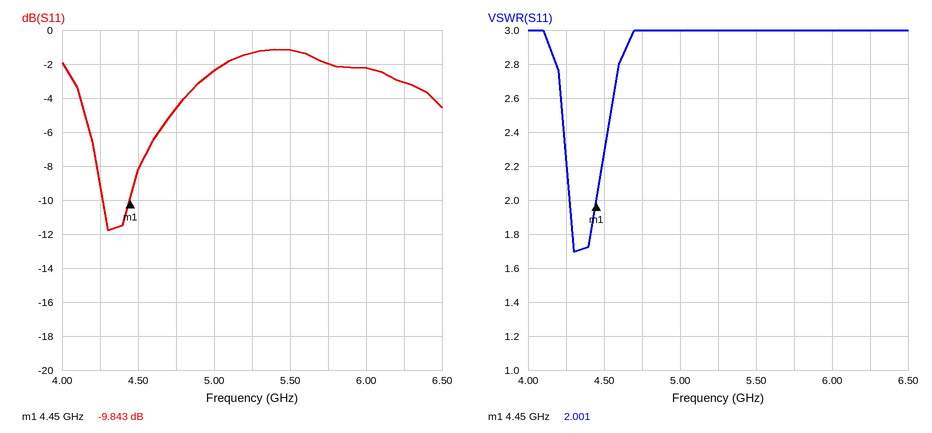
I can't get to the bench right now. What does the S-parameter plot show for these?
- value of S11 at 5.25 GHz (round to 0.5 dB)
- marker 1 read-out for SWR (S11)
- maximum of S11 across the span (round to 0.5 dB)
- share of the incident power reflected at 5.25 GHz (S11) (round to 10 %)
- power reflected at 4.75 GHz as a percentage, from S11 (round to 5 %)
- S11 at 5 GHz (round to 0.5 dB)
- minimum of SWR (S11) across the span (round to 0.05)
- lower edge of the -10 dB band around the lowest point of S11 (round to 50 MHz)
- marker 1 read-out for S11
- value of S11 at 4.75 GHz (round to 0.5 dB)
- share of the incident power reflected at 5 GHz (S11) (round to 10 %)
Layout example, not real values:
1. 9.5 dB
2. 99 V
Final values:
1. -1.5 dB
2. 2.001
3. -1.0 dB
4. 70 %
5. 35 %
6. -2.5 dB
7. 1.70
8. 4.25 GHz
9. -9.843 dB
10. -4.5 dB
11. 60 %
